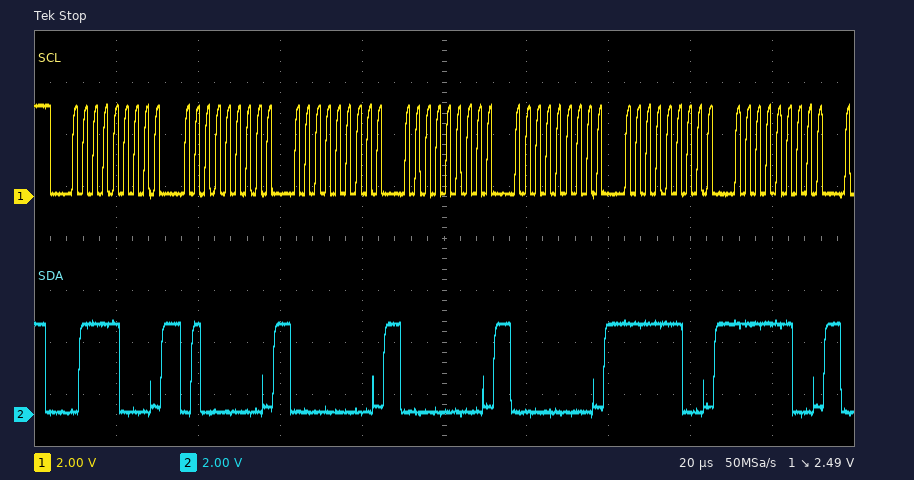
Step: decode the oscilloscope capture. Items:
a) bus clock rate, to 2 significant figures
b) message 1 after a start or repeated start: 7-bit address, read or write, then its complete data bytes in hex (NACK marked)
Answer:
400 kHz
0x3C write: 40 00 00 00 FC FC
